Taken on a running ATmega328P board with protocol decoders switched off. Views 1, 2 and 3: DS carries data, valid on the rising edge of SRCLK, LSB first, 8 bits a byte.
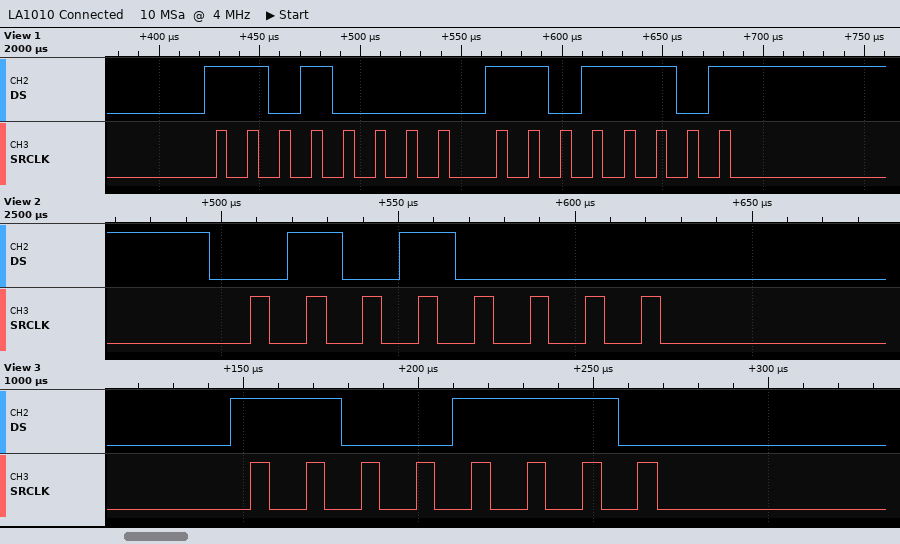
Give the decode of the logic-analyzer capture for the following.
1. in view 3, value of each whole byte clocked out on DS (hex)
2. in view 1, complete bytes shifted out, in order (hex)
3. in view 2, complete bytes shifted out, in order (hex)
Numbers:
73
0B BB
0A
